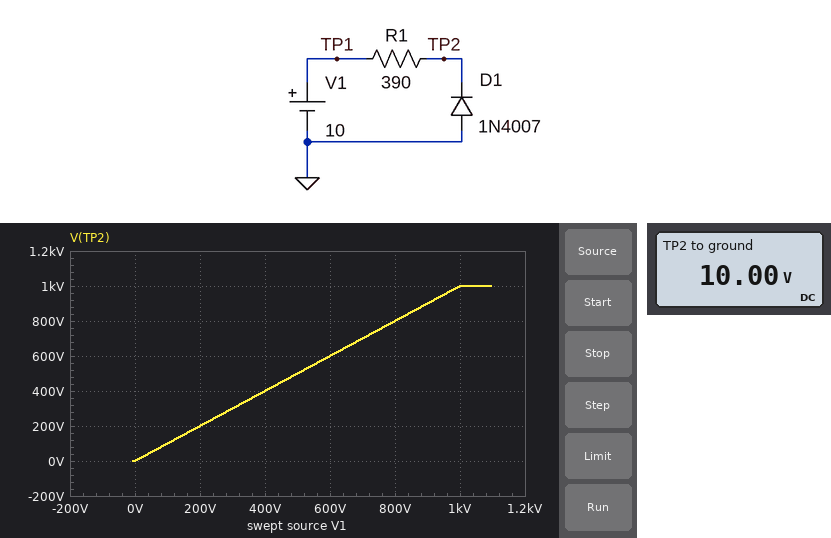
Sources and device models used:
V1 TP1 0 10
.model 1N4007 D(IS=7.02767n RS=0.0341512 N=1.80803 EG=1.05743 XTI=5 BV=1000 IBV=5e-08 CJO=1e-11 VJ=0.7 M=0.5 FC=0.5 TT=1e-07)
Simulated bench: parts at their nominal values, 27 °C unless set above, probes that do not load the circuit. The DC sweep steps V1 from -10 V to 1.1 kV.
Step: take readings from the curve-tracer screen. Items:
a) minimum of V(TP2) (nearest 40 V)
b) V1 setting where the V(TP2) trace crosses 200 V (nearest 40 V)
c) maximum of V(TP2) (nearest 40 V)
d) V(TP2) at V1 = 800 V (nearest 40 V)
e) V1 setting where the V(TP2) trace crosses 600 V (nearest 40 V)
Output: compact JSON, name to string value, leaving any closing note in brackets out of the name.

{"minimum of V(TP2)": "0 V", "V1 setting where the V(TP2) trace crosses 200 V": "200 V", "maximum of V(TP2)": "1.00 kV", "V(TP2) at V1 = 800 V": "800 V", "V1 setting where the V(TP2) trace crosses 600 V": "600 V"}
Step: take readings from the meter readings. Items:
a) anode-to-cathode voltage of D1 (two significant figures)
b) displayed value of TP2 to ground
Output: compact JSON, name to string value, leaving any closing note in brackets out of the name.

{"anode-to-cathode voltage of D1": "-10 V", "displayed value of TP2 to ground": "10.00 V"}
